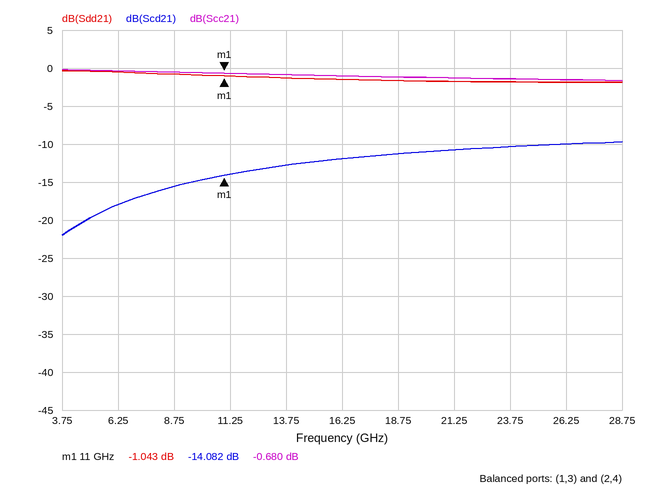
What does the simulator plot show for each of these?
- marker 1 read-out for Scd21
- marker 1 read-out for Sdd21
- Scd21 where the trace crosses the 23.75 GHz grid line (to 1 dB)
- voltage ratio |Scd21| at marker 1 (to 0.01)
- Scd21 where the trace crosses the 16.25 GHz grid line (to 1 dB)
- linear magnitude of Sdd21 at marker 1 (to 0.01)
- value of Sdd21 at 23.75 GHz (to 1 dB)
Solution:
-14.082 dB
-1.043 dB
-10 dB
0.20
-12 dB
0.89
-2 dB
